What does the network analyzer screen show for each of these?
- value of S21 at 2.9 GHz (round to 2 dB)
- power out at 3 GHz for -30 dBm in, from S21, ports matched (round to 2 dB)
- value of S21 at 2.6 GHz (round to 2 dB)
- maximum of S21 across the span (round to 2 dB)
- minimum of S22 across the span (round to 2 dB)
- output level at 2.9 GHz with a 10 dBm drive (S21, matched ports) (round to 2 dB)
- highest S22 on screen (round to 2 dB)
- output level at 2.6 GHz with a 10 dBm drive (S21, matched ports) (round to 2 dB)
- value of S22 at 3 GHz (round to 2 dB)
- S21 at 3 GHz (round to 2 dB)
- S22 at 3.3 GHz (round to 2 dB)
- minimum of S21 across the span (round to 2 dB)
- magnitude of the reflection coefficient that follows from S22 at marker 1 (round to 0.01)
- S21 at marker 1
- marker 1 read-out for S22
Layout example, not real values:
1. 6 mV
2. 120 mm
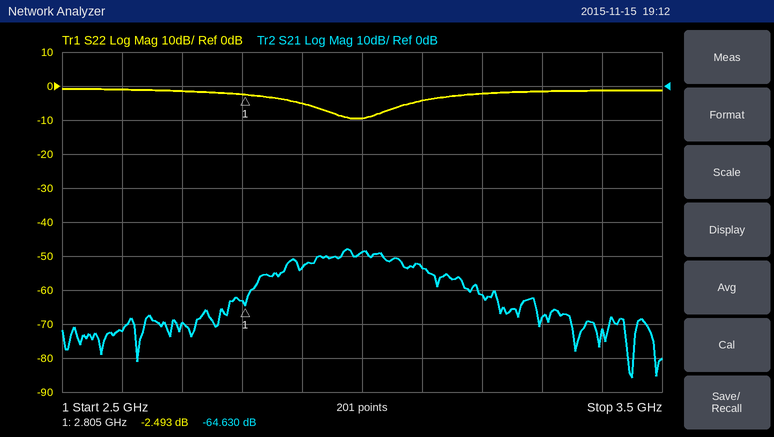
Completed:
1. -54 dB
2. -78 dBm
3. -72 dB
4. -48 dB
5. -10 dB
6. -44 dBm
7. 0 dB
8. -62 dBm
9. -10 dB
10. -48 dB
11. -2 dB
12. -86 dB
13. 0.75
14. -64.630 dB
15. -2.493 dB
